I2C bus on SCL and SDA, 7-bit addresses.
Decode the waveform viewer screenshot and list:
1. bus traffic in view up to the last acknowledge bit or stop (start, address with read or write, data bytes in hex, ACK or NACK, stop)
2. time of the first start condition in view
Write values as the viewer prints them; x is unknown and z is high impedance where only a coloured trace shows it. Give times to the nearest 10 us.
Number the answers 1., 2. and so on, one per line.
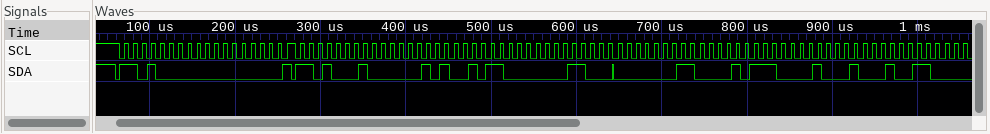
1. start, address 68 write ACK, 00 ACK, repeated start, address 68 read ACK, 05 ACK, 58 ACK, 18 ACK, 03 ACK, 17 ACK, 11 ACK, 26 ACK
2. 60 us
